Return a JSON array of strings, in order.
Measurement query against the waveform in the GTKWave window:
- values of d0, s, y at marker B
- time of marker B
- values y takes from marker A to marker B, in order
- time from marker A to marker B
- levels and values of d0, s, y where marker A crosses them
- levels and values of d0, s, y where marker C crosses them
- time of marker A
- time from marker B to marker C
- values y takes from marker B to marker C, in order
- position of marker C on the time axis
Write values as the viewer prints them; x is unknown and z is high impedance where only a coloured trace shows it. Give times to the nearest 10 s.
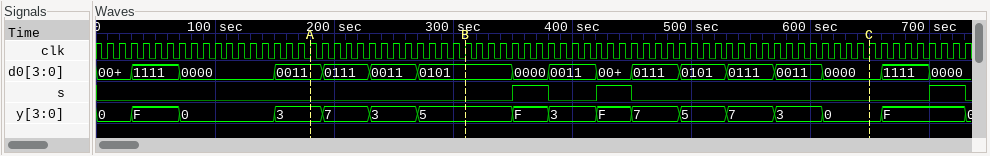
["d0=0101, s=0, y=5", "310 s", "3, 7, 3, 5", "130 s", "d0=0011, s=0, y=3", "d0=0000, s=0, y=0", "180 s", "340 s", "5, F, 3, F, 7, 5, 7, 3, 0", "650 s"]
